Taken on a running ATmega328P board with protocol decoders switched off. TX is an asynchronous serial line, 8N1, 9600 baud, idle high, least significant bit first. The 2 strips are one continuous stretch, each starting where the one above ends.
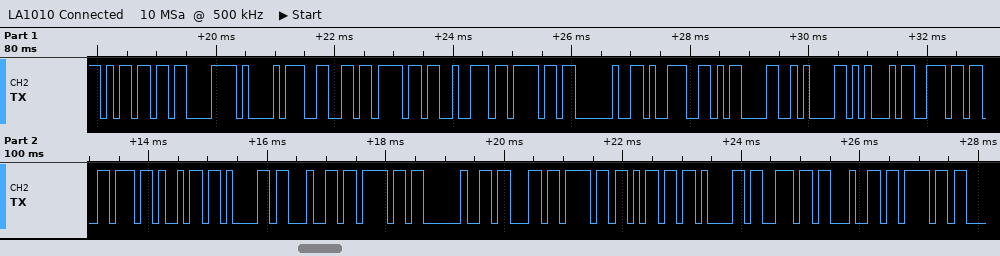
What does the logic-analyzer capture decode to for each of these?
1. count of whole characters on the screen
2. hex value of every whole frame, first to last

26
6D C3 A1 66 6F 72 6F 20 39 0D 0A 45 6E 76 69 61 64 6F 20 63 6F 6D 61 6E 64 6F
